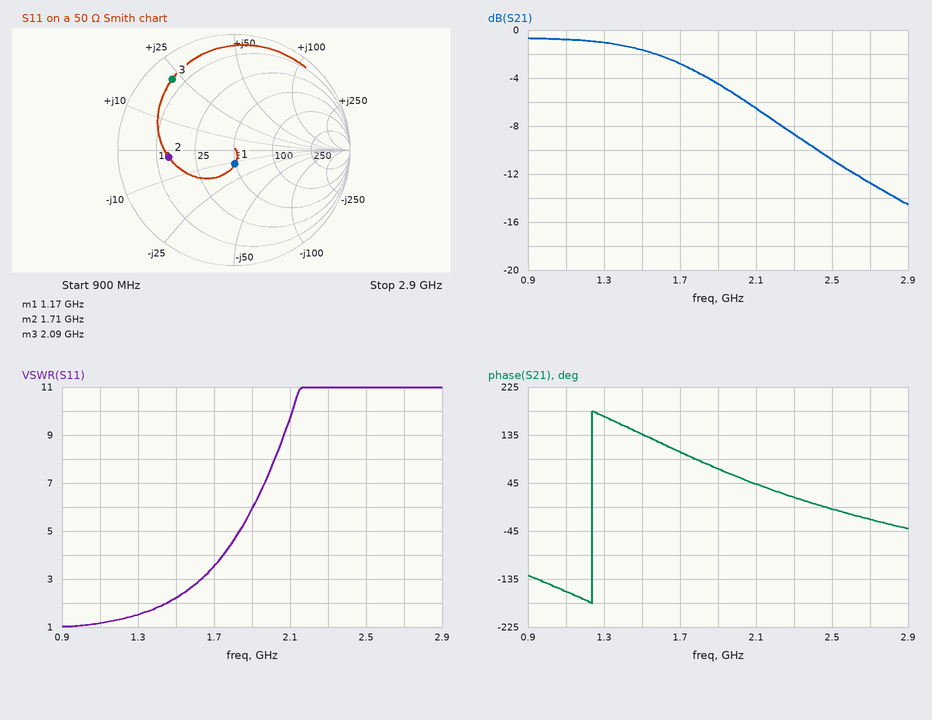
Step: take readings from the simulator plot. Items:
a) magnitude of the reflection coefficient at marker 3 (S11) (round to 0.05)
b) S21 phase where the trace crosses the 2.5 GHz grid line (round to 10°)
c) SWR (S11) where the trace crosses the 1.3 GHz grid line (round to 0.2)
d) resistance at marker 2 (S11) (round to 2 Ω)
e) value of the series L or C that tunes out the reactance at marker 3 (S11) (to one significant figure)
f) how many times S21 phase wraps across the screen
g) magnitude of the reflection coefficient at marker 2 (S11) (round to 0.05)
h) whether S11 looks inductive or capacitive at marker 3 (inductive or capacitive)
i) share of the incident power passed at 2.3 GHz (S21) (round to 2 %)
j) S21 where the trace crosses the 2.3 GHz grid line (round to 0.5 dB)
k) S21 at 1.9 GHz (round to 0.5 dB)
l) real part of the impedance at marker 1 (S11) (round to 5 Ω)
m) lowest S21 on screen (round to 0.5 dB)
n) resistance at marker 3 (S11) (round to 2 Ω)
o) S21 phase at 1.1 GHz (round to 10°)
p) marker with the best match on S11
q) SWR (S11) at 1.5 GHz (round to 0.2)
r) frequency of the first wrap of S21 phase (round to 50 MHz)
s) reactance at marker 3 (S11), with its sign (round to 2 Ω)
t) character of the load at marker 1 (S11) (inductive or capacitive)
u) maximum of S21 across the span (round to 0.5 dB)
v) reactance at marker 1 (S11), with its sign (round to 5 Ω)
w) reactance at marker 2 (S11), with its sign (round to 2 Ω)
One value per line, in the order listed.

0.80
0°
1.6
14 Ω
3 pF
1
0.55
inductive
14 %
-8.5 dB
-4.5 dB
50 Ω
-14.5 dB
6 Ω
-160°
marker 1
2.2
1.25 GHz
+22 Ω
capacitive
-0.5 dB
-10 Ω
-2 Ω
